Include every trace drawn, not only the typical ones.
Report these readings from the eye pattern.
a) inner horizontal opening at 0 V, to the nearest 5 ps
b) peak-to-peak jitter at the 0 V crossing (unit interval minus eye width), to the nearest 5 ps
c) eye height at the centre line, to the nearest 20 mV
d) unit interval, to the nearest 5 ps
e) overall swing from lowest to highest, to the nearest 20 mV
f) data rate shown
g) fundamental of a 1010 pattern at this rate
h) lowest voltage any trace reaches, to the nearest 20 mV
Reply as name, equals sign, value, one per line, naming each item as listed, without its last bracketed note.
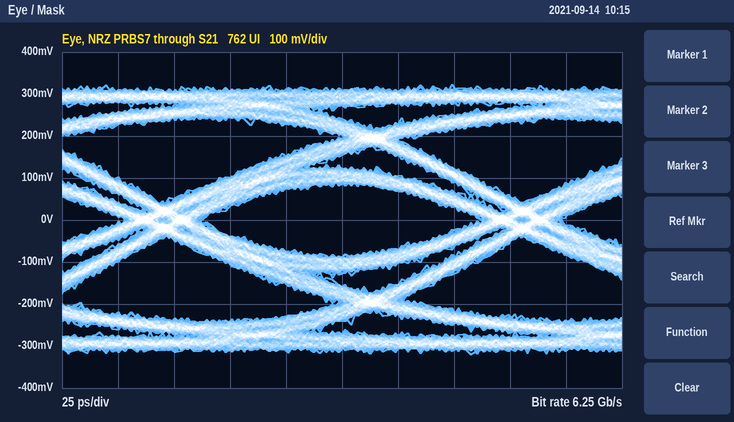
inner horizontal opening at 0 V, to the nearest 5 ps = 125 ps
peak-to-peak jitter at the 0 V crossing (unit interval minus eye width), to the nearest 5 ps = 35 ps
eye height at the centre line, to the nearest 20 mV = 180 mV
unit interval, to the nearest 5 ps = 160 ps
overall swing from lowest to highest, to the nearest 20 mV = 640 mV
data rate shown = 6.25 Gb/s
fundamental of a 1010 pattern at this rate = 3.125 GHz
lowest voltage any trace reaches, to the nearest 20 mV = -320 mV
